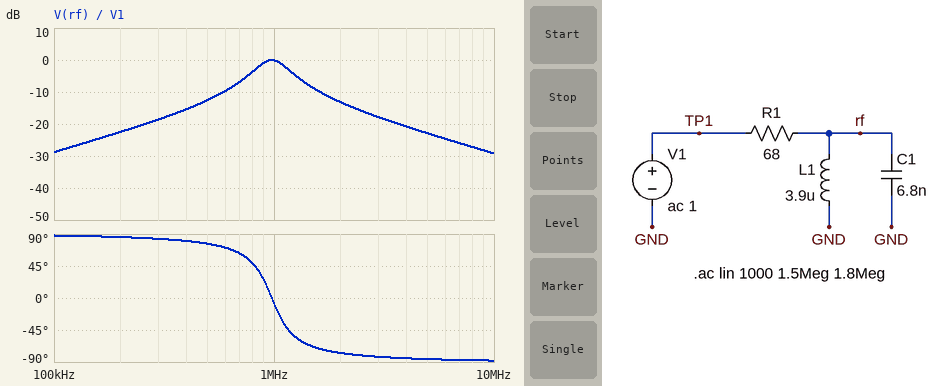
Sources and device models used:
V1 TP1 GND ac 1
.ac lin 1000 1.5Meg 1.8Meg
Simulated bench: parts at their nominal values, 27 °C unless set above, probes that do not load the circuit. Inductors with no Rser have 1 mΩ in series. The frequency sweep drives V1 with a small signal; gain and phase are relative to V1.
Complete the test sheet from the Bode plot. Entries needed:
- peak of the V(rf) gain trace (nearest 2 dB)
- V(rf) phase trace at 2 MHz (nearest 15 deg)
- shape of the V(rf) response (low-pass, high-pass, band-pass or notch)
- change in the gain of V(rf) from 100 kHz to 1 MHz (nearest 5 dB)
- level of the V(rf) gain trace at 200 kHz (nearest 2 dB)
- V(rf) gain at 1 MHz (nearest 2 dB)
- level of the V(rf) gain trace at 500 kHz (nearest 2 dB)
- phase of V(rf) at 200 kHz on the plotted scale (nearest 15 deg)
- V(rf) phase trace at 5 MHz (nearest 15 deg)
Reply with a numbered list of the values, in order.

1. 0 dB
2. -75 deg
3. band-pass
4. 30 dB
5. -22 dB
6. 0 dB
7. -12 dB
8. 90 deg
9. -90 deg
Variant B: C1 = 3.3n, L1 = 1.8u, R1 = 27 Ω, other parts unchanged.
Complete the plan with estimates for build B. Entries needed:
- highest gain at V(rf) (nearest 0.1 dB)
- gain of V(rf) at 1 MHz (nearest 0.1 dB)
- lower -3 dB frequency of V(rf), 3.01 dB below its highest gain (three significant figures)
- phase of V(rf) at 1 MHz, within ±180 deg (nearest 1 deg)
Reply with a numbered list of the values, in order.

1. 0 dB
2. -6.4 dB
3. 1.36 MHz
4. 61 deg
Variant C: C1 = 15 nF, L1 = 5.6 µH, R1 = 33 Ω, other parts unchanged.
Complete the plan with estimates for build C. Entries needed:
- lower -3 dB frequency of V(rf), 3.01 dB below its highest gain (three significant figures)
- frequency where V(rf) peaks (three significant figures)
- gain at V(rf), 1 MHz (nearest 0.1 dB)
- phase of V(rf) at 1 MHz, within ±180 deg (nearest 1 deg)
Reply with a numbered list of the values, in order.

1. 411 kHz
2. 549 kHz
3. -7.6 dB
4. -65 deg
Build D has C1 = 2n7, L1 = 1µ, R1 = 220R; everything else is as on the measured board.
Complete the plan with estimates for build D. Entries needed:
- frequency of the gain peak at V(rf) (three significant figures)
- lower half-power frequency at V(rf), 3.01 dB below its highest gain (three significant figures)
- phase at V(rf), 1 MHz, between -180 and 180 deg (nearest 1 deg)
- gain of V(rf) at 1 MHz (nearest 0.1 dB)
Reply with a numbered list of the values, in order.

1. 3.06 MHz
2. 2.93 MHz
3. 88 deg
4. -29.9 dB
